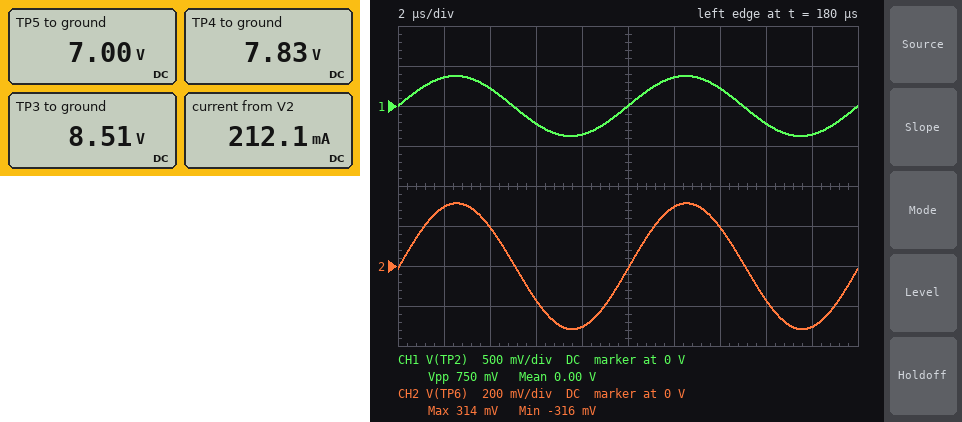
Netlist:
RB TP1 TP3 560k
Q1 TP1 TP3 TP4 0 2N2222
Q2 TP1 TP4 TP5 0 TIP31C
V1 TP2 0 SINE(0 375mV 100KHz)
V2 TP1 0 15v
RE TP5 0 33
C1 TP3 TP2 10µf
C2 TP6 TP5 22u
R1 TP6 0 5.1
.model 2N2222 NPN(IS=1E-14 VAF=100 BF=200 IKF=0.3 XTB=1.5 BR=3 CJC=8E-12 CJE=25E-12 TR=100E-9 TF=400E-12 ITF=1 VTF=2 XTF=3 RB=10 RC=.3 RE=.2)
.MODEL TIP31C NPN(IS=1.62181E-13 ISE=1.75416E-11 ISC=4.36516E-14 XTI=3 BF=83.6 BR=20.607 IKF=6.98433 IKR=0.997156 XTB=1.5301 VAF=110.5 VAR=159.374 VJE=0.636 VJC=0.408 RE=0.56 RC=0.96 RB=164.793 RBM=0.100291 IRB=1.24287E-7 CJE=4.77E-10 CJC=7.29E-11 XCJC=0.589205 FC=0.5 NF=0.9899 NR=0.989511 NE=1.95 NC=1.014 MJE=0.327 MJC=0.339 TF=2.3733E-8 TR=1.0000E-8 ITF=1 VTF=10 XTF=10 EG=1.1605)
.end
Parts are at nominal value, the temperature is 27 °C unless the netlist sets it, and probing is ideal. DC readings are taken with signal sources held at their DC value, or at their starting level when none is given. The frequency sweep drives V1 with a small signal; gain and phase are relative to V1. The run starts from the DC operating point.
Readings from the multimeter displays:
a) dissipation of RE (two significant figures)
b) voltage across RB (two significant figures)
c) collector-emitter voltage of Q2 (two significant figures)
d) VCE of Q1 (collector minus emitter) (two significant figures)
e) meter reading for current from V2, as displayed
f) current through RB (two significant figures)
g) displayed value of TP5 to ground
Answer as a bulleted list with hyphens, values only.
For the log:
- 1.5 W
- 6.5 V
- 8.0 V
- 7.2 V
- 212.1 mA
- 12 µA
- 7.00 V
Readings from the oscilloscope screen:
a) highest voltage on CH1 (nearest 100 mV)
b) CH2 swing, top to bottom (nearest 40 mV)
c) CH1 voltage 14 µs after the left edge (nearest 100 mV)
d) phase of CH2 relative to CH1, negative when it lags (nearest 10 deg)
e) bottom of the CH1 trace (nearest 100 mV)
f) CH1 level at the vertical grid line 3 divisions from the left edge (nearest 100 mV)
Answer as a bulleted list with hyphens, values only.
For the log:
- 400 mV
- 640 mV
- 200 mV
- 0 deg
- -400 mV
- -200 mV
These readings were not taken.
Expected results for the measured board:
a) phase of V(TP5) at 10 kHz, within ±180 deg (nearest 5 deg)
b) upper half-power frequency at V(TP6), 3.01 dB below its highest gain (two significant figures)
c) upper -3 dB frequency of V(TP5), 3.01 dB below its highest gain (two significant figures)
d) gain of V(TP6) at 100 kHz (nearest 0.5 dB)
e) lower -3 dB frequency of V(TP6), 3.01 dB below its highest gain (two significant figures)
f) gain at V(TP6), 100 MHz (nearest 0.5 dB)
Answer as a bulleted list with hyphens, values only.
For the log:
- 0 deg
- 1.6 MHz
- 1.1 MHz
- -1.5 dB
- 1.2 kHz
- -11.5 dB
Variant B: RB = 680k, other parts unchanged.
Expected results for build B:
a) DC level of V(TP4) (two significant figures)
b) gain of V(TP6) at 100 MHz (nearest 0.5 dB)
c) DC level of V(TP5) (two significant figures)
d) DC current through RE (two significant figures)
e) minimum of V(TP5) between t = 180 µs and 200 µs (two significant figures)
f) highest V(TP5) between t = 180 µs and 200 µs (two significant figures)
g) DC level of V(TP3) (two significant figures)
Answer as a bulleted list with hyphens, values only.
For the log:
- 7.2 V
- -12.0 dB
- 6.4 V
- 190 mA
- 6.1 V
- 6.7 V
- 7.9 V
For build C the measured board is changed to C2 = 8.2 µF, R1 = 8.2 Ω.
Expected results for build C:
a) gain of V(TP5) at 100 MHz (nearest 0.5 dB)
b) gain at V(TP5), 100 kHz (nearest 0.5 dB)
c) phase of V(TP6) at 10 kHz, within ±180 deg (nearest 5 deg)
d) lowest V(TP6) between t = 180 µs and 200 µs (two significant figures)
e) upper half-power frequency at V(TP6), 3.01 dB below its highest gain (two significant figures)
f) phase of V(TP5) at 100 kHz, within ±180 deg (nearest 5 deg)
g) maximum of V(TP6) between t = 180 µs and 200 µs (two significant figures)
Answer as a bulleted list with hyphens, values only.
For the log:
- -9.5 dB
- -1.0 dB
- 10 deg
- -330 mV
- 2.1 MHz
- 0 deg
- 330 mV
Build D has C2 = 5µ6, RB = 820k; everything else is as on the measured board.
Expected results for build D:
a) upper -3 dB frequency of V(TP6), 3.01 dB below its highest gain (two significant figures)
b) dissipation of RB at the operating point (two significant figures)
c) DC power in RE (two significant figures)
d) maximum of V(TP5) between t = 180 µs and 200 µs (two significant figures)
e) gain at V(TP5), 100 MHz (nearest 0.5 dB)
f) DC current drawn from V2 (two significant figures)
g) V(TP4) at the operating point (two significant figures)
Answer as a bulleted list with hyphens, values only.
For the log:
- 1.5 MHz
- 72 µW
- 1.0 W
- 6.1 V
- -12.5 dB
- 180 mA
- 6.6 V
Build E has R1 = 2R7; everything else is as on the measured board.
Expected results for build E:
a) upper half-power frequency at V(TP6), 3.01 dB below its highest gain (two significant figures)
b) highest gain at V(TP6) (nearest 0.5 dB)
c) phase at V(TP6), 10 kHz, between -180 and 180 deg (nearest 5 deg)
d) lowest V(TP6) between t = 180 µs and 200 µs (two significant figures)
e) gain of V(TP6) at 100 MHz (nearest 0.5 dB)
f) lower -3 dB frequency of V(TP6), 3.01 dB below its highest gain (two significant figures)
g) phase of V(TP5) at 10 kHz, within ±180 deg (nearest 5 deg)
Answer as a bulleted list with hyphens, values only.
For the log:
- 1.1 MHz
- -2.5 dB
- 10 deg
- -280 mV
- -15.5 dB
- 2.1 kHz
- -5 deg
